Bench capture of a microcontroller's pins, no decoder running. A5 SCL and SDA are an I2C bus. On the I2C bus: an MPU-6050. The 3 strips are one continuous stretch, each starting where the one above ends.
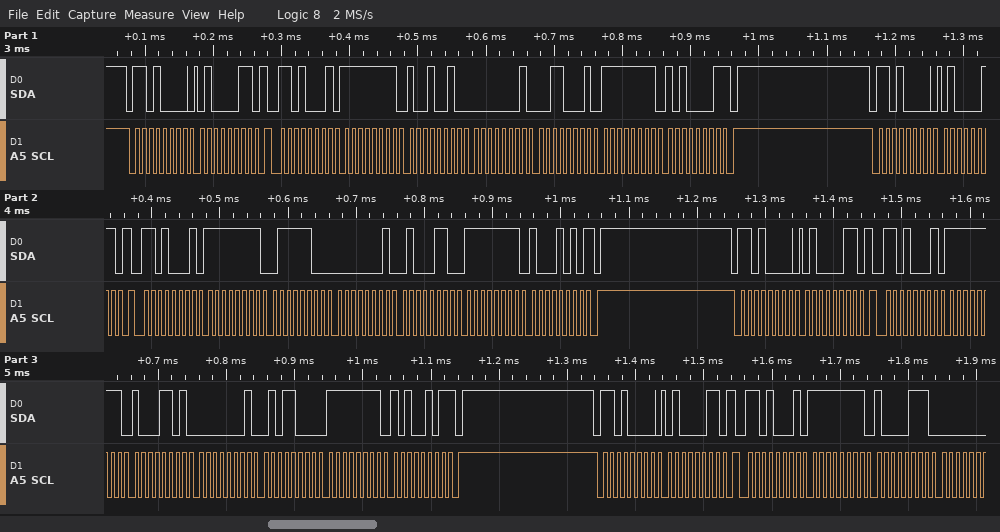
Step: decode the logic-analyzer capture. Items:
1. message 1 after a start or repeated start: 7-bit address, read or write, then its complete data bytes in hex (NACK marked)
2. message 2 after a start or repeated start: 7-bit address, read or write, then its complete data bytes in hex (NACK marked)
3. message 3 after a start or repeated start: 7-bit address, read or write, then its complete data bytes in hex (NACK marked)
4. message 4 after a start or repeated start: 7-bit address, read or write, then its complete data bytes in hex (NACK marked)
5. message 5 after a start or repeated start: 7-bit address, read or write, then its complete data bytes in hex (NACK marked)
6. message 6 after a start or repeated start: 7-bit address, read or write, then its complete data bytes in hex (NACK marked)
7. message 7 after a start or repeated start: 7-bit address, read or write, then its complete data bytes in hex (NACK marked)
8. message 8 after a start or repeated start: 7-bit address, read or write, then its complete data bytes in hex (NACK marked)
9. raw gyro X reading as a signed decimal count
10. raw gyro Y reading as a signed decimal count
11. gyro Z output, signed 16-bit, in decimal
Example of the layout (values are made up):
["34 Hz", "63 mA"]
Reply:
["0x68 write: 43", "0x68 read: FF 92 01 31 FF A1 NACK", "0x68 write: 43", "0x68 read: FF 7C 01 46 FF 8A NACK", "0x68 write: 43", "0x68 read: FF 8D 01 58 FF A5 NACK", "0x68 write: 43", "0x68 read: FF 87", "-110", "305", "-95"]
